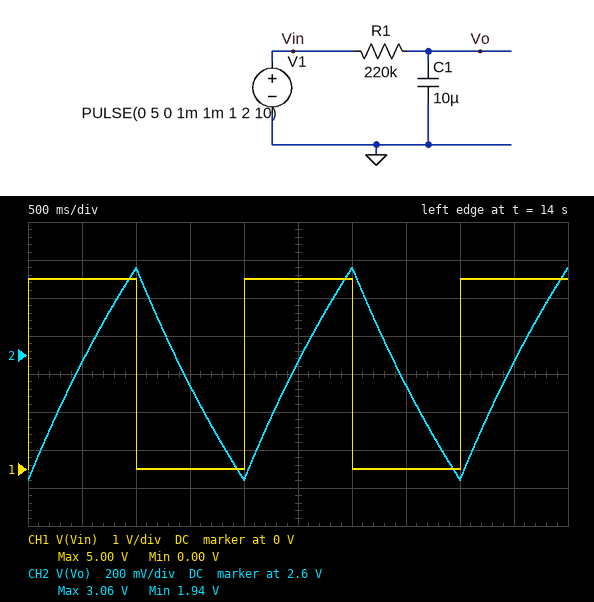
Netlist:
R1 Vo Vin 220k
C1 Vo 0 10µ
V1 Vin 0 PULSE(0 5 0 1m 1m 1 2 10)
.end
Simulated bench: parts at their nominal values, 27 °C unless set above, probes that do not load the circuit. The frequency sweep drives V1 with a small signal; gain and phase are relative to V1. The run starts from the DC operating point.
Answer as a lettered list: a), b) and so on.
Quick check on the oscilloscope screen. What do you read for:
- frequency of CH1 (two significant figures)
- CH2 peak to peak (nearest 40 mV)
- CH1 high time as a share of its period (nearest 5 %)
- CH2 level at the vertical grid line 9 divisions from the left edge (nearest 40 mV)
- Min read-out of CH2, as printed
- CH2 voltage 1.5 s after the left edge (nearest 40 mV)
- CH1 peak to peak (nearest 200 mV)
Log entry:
a) 500 mHz
b) 1.12 V
c) 50 %
d) 2.56 V
e) 1.94 V
f) 2.44 V
g) 5.0 V
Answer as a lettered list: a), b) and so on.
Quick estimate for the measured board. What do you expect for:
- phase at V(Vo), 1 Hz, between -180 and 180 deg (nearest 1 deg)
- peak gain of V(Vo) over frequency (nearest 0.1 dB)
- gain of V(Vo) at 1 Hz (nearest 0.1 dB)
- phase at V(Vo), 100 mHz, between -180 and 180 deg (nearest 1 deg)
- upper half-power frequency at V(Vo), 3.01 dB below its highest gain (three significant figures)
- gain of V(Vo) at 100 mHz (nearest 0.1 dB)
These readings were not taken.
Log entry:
a) -86 deg
b) 0 dB
c) -22.8 dB
d) -54 deg
e) 72.3 mHz
f) -4.6 dB
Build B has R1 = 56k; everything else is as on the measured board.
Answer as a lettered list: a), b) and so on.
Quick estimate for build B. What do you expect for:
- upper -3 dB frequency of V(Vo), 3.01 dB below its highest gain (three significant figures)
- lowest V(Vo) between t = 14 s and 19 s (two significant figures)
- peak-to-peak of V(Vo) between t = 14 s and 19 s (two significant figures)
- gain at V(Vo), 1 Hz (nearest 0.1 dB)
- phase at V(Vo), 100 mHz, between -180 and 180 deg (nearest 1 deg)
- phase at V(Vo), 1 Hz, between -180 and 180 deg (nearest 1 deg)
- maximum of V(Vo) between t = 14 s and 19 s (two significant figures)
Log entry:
a) 284 mHz
b) 720 mV
c) 3.6 V
d) -11.3 dB
e) -19 deg
f) -74 deg
g) 4.3 V
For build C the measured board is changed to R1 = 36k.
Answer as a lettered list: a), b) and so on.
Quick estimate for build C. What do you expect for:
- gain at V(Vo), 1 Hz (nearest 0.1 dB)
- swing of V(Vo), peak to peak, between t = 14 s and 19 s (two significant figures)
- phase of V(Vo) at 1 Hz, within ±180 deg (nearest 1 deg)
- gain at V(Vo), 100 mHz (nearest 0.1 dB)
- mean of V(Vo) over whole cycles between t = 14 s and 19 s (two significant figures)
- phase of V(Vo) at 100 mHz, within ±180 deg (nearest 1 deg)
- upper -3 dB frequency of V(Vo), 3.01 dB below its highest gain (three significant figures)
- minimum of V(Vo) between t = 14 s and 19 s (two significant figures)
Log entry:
a) -7.9 dB
b) 4.4 V
c) -66 deg
d) -0.2 dB
e) 2.5 V
f) -13 deg
g) 442 mHz
h) 290 mV
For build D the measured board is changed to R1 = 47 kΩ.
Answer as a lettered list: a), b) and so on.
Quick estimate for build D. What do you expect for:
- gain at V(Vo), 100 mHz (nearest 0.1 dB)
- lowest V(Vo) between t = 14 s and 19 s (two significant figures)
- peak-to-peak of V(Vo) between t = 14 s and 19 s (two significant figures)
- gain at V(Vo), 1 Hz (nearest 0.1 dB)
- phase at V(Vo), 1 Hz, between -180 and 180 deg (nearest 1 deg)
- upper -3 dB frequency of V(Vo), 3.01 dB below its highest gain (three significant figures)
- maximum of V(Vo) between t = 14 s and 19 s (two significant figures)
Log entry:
a) -0.4 dB
b) 530 mV
c) 3.9 V
d) -9.9 dB
e) -71 deg
f) 339 mHz
g) 4.5 V
